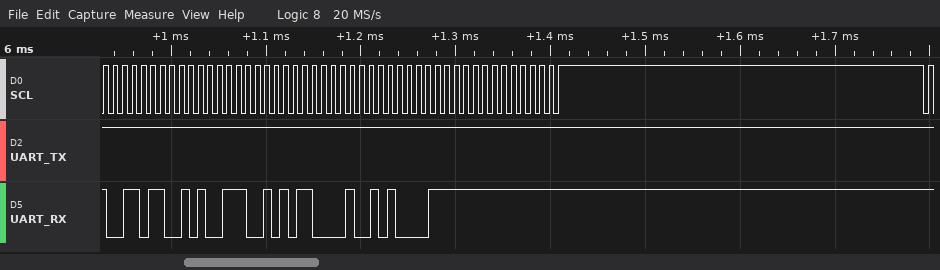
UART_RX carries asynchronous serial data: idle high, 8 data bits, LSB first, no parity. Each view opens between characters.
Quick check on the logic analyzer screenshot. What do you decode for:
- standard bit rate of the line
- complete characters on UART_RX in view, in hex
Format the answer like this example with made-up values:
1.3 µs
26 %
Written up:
115200 baud
36, 39, 0D, 0A
